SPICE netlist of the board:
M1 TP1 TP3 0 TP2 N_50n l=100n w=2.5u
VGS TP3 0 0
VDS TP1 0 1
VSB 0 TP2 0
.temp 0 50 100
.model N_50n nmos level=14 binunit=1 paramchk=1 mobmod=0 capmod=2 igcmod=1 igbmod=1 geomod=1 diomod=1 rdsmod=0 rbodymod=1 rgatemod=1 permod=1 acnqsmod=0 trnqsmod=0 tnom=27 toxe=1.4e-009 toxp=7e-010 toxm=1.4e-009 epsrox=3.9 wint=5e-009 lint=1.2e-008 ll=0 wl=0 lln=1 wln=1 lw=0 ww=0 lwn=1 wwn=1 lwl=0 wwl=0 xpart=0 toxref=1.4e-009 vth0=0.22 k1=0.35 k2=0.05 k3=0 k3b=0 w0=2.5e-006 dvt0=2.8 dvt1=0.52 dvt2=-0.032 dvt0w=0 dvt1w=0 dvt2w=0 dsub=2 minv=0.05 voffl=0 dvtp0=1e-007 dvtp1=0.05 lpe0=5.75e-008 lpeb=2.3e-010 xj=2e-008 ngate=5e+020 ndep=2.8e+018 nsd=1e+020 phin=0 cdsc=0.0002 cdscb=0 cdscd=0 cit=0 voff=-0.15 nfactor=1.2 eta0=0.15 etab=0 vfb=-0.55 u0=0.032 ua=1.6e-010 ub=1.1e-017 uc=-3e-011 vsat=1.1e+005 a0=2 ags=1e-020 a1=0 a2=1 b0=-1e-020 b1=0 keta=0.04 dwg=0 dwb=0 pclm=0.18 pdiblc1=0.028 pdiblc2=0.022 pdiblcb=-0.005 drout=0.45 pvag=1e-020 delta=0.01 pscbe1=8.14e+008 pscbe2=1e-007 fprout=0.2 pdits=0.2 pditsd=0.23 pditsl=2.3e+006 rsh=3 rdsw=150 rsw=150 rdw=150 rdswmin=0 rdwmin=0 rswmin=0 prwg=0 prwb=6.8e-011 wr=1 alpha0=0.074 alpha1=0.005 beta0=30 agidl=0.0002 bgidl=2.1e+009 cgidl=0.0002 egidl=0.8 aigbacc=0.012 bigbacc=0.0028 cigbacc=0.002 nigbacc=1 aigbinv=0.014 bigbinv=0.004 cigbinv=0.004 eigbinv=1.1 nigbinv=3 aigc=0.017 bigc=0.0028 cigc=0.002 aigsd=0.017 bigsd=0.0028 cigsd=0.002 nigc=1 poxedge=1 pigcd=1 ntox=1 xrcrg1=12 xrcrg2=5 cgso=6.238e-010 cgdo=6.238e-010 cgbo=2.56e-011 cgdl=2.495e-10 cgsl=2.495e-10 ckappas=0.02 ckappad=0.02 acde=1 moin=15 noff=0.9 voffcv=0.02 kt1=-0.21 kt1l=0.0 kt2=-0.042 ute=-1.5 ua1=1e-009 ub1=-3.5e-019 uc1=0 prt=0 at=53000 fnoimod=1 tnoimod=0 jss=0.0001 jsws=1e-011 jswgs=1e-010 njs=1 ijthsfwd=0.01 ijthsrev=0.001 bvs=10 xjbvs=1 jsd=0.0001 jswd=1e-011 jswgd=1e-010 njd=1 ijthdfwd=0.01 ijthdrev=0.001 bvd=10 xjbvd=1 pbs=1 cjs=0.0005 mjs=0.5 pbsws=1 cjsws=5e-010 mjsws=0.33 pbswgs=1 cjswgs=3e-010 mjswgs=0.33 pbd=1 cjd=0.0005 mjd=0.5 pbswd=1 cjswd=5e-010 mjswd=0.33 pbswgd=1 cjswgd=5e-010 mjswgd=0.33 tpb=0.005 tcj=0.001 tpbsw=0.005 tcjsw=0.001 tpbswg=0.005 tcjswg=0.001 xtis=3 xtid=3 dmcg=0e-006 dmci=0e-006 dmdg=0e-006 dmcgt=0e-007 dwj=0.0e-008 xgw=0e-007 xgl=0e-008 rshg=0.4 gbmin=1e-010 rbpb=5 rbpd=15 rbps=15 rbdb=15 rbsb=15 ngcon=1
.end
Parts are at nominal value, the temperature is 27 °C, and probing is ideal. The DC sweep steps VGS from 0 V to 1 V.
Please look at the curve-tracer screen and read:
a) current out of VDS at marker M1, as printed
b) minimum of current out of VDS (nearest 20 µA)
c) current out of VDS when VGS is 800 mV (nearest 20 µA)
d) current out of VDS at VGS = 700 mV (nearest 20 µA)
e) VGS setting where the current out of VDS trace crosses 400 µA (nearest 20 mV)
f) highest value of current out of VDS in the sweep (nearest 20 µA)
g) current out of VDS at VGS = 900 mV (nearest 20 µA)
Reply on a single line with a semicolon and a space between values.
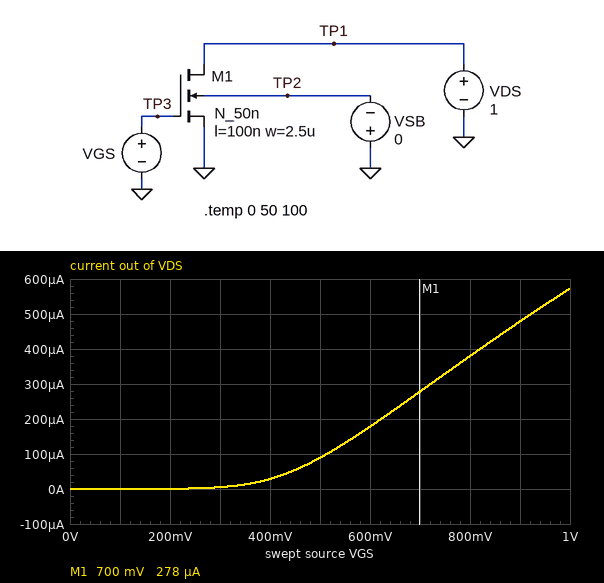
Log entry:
278 µA; 0 A; 380 µA; 280 µA; 820 mV; 580 µA; 480 µA
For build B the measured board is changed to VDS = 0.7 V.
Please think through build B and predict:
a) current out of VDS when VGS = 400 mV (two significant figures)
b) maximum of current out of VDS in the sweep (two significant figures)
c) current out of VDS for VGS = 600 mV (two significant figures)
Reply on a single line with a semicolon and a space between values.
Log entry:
25 µA; 540 µA; 170 µA
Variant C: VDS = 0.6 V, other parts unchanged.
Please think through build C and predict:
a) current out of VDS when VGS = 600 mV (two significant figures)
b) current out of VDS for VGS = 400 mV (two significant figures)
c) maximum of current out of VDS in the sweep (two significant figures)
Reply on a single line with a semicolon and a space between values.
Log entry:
160 µA; 24 µA; 530 µA
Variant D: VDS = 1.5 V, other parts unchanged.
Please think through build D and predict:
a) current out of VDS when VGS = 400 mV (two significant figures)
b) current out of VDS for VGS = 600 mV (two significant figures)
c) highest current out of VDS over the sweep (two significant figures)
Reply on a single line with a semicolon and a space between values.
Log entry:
35 µA; 200 µA; 620 µA
